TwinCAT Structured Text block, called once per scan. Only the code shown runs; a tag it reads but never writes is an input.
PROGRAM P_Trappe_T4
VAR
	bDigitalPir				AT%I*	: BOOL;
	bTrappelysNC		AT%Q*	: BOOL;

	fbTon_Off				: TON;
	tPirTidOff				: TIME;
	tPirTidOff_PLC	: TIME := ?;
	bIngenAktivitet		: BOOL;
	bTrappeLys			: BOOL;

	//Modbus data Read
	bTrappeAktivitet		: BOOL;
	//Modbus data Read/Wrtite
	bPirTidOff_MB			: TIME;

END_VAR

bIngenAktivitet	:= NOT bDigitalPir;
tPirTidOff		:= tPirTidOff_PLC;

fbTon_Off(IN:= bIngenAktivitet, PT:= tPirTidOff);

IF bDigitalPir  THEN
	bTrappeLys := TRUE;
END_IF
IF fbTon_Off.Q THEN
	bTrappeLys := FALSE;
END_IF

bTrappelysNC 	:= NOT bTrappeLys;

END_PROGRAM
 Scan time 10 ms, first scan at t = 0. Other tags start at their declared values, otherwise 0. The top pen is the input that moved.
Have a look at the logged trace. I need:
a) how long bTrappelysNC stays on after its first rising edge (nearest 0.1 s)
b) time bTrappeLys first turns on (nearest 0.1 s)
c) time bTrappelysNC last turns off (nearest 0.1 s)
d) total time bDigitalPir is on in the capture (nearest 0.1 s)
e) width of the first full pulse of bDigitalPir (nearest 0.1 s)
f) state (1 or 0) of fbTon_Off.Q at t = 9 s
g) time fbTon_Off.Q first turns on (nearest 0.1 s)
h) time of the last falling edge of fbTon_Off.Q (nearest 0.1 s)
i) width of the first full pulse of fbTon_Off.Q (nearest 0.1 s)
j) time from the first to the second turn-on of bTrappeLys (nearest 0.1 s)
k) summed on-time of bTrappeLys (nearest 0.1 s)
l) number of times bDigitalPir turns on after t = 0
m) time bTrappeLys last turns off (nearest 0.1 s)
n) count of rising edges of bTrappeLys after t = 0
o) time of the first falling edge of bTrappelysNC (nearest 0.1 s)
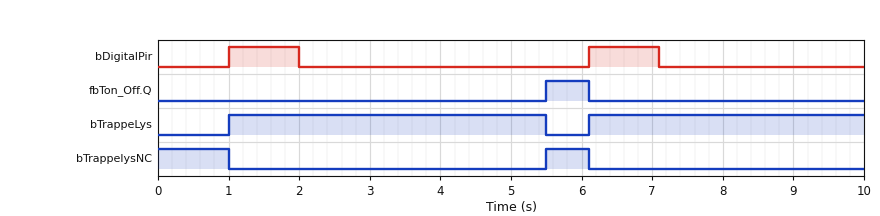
0.6 s
1.0 s
6.1 s
2.0 s
1.0 s
0
5.5 s
6.1 s
0.6 s
5.1 s
8.4 s
2
5.5 s
2
1.0 s
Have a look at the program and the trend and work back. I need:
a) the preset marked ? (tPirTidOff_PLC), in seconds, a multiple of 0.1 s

3.5 s
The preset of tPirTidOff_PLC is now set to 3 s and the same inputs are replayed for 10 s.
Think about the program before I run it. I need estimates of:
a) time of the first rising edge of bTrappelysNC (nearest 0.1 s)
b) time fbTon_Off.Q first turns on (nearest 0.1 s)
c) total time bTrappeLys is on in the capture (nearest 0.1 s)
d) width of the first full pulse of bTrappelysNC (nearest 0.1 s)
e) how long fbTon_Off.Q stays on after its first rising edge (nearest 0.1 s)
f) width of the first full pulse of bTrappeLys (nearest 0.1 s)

5.0 s
5.0 s
7.9 s
1.1 s
1.1 s
4.0 s
